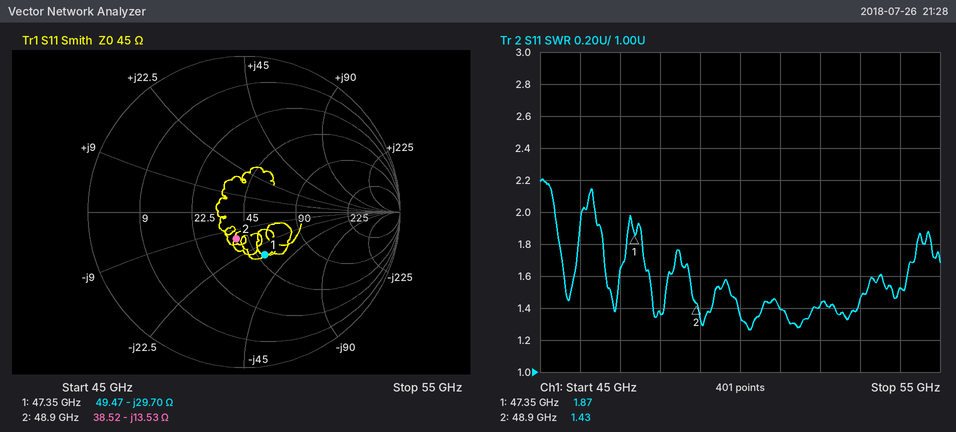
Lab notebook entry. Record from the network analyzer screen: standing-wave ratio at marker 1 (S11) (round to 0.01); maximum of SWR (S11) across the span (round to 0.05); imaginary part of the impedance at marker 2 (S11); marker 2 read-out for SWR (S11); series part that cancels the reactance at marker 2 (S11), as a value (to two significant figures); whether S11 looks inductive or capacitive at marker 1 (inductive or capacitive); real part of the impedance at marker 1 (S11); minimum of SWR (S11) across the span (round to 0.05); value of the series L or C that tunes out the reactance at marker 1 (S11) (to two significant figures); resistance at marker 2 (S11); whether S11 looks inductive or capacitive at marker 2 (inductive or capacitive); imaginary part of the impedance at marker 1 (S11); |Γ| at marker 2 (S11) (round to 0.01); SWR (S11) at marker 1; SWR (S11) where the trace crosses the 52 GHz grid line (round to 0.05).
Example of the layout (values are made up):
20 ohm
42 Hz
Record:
1.87
2.20
-13.53 Ω
1.43
44 pH
capacitive
49.47 Ω
1.25
100 pH
38.52 Ω
capacitive
-29.70 Ω
0.18
1.87
1.40
